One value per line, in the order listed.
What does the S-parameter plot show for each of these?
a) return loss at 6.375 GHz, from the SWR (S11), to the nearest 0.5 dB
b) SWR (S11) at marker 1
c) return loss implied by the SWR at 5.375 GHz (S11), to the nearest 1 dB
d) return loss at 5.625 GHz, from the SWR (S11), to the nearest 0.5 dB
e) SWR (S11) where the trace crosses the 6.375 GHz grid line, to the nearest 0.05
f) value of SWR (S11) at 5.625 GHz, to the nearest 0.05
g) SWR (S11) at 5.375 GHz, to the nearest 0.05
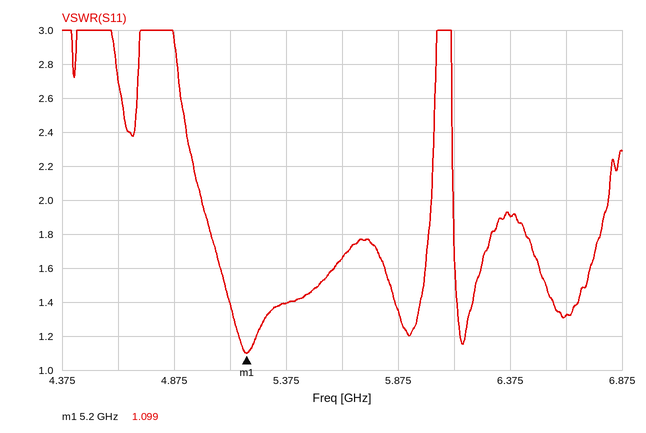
10.0 dB
1.099
16 dB
12.0 dB
1.90
1.65
1.40
